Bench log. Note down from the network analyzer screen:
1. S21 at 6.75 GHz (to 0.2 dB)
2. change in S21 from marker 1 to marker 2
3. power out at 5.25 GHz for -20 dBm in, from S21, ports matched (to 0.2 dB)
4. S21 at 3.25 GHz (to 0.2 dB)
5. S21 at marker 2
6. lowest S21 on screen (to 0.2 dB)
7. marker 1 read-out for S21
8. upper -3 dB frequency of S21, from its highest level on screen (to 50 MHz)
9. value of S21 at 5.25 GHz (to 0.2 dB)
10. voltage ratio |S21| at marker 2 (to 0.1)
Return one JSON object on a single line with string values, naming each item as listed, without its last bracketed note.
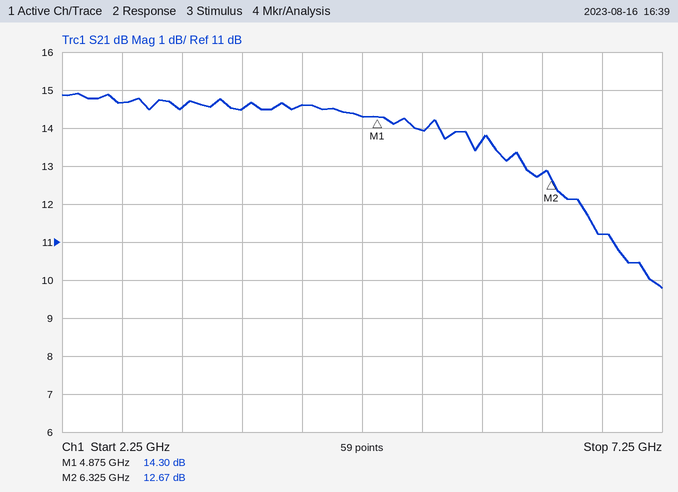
{"S21 at 6.75 GHz": "11.2 dB", "change in S21 from marker 1 to marker 2": "-1.63 dB", "power out at 5.25 GHz for -20 dBm in, from S21, ports matched": "-6.0 dBm", "S21 at 3.25 GHz": "14.6 dB", "S21 at marker 2": "12.67 dB", "lowest S21 on screen": "9.8 dB", "marker 1 read-out for S21": "14.30 dB", "upper -3 dB frequency of S21, from its highest level on screen": "6.60 GHz", "value of S21 at 5.25 GHz": "14.0 dB", "voltage ratio |S21| at marker 2": "4.3"}
